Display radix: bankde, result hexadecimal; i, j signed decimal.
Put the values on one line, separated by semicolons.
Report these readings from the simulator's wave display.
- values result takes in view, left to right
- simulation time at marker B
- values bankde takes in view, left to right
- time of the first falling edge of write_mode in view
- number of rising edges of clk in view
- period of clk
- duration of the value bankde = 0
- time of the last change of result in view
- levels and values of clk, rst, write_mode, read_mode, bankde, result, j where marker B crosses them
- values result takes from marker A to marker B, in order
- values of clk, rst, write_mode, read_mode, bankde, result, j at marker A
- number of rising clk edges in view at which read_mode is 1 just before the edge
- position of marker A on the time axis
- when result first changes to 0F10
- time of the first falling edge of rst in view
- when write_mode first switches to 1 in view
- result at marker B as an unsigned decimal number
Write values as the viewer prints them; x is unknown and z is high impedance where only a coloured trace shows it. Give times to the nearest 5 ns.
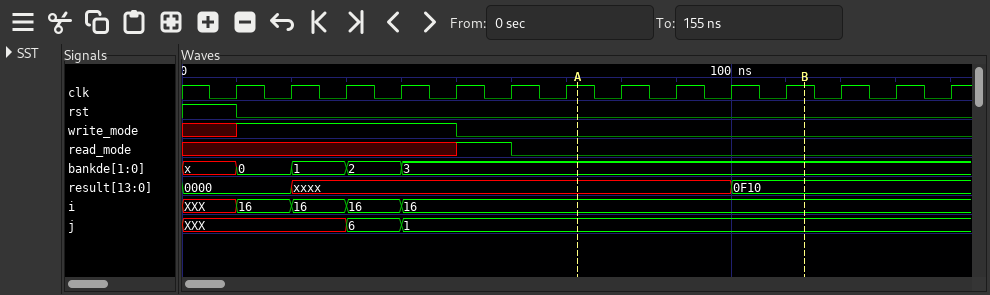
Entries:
0000, xxxx, 0F10; 115 ns; x, 0, 1, 2, 3; 50 ns; 14; 10 ns; 10 ns; 100 ns; clk=1, rst=0, write_mode=0, read_mode=0, bankde=3, result=0F10, j=1; xxxx, 0F10; clk=1, rst=0, write_mode=0, read_mode=0, bankde=3, result=xxxx, j=1; 1; 70 ns; 100 ns; 10 ns; 10 ns; 3856
